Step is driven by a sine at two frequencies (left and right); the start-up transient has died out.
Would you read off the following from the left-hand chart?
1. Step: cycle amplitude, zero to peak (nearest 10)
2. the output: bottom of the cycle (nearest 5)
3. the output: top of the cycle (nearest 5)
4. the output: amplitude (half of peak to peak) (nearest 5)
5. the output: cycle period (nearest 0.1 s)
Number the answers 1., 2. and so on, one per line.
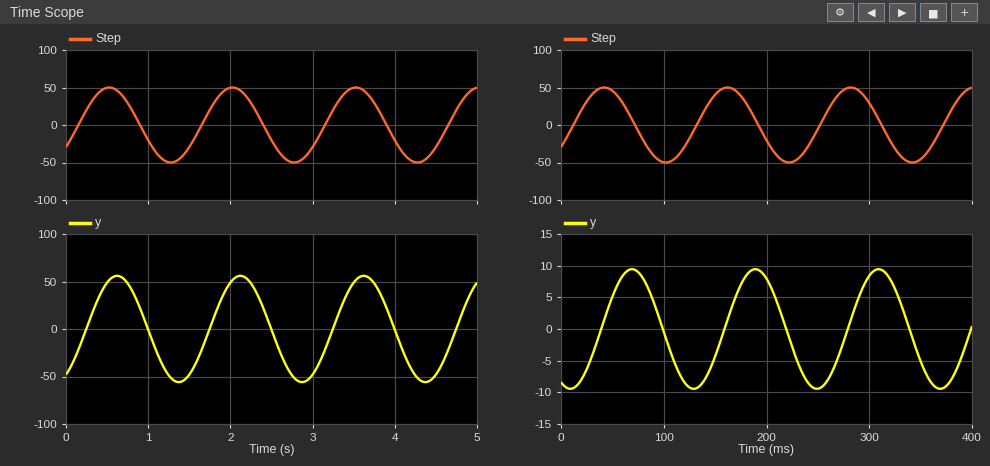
1. 50
2. -55
3. 55
4. 55
5. 1.5 s
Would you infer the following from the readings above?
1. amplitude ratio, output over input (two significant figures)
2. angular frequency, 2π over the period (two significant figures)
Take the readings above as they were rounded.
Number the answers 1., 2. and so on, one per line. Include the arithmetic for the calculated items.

1. 55 / 50 = 1.1
2. 2π / 1.5 = 4.2 rad/s
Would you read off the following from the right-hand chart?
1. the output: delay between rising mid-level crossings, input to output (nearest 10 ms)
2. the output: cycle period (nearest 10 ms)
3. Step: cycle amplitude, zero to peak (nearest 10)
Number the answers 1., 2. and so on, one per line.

1. 30 ms
2. 120 ms
3. 50
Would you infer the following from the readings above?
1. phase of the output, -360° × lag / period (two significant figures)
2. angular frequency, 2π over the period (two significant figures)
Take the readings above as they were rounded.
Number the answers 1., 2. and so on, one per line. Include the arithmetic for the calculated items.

1. -360 × 30 / 120 = -90°
2. 2π / 120 = 0.052 rad/ms
